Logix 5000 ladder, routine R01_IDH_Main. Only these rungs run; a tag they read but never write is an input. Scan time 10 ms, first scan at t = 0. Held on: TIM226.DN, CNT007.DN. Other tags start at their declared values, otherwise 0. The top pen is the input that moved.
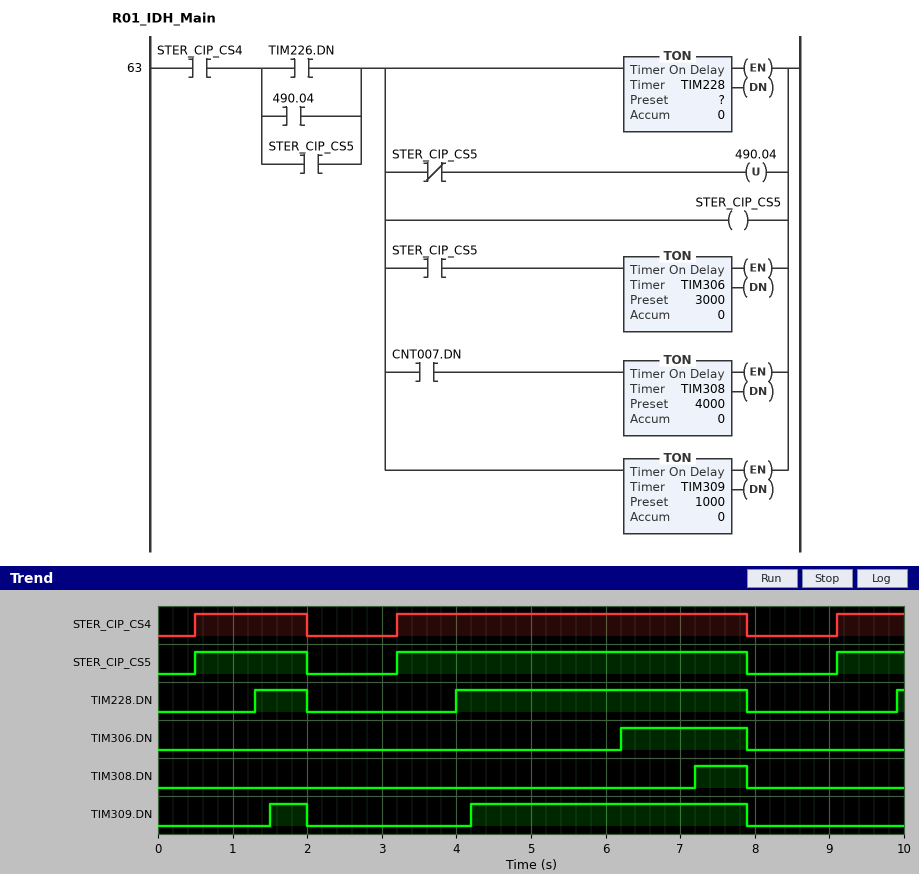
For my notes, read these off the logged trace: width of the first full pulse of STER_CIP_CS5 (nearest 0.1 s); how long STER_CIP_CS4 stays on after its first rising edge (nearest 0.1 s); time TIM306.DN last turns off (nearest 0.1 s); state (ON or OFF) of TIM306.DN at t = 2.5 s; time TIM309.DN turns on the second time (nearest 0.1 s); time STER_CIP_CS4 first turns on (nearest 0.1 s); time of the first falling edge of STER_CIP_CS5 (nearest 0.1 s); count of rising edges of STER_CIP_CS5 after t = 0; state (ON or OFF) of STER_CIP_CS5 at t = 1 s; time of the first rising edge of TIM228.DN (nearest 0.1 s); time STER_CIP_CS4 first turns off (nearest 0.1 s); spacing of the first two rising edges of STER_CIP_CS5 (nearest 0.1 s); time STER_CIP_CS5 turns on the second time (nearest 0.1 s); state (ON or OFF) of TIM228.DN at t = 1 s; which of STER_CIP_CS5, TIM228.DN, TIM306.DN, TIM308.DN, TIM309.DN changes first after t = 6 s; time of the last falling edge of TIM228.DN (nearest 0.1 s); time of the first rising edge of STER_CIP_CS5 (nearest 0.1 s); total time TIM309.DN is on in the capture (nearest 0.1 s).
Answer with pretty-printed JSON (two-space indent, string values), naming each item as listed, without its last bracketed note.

{
  "width of the first full pulse of STER_CIP_CS5": "1.5 s",
  "how long STER_CIP_CS4 stays on after its first rising edge": "1.5 s",
  "time TIM306.DN last turns off": "7.9 s",
  "state (ON or OFF) of TIM306.DN at t = 2.5 s": "OFF",
  "time TIM309.DN turns on the second time": "4.2 s",
  "time STER_CIP_CS4 first turns on": "0.5 s",
  "time of the first falling edge of STER_CIP_CS5": "2.0 s",
  "count of rising edges of STER_CIP_CS5 after t = 0": "3",
  "state (ON or OFF) of STER_CIP_CS5 at t = 1 s": "ON",
  "time of the first rising edge of TIM228.DN": "1.3 s",
  "time STER_CIP_CS4 first turns off": "2.0 s",
  "spacing of the first two rising edges of STER_CIP_CS5": "2.7 s",
  "time STER_CIP_CS5 turns on the second time": "3.2 s",
  "state (ON or OFF) of TIM228.DN at t = 1 s": "OFF",
  "which of STER_CIP_CS5, TIM228.DN, TIM306.DN, TIM308.DN, TIM309.DN changes first after t = 6 s": "TIM306.DN",
  "time of the last falling edge of TIM228.DN": "7.9 s",
  "time of the first rising edge of STER_CIP_CS5": "0.5 s",
  "total time TIM309.DN is on in the capture": "4.2 s"
}
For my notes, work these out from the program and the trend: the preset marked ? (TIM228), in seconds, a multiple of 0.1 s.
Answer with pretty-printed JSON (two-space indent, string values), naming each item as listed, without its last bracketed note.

{
  "the preset marked ? (TIM228), in seconds, a multiple of 0.1 s": "0.8 s"
}
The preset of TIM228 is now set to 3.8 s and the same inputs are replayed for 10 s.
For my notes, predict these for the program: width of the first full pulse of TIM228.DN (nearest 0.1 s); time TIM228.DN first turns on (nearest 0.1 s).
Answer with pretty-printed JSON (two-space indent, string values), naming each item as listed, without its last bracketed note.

{
  "width of the first full pulse of TIM228.DN": "0.9 s",
  "time TIM228.DN first turns on": "7.0 s"
}
